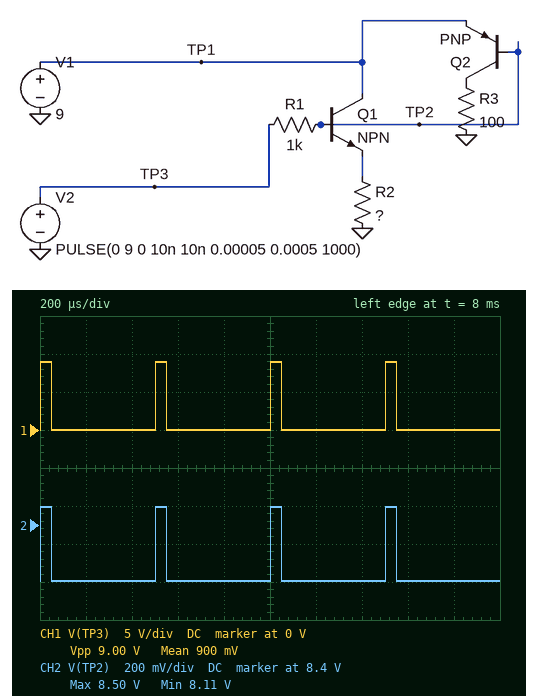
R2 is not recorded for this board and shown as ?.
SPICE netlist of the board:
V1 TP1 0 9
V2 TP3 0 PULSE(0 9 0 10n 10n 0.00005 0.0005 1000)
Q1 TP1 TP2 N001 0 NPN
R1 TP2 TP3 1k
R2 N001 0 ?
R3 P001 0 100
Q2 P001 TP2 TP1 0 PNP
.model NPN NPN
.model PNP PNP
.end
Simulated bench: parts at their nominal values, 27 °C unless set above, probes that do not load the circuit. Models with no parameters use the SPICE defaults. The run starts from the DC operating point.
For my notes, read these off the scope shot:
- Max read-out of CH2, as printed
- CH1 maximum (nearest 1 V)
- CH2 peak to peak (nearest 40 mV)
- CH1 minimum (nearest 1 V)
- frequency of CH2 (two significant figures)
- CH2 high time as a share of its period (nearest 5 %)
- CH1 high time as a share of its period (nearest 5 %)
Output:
8.50 V
9 V
400 mV
0 V
2.0 kHz
10 %
10 %
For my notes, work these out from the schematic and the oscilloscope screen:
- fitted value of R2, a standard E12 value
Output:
150 Ω
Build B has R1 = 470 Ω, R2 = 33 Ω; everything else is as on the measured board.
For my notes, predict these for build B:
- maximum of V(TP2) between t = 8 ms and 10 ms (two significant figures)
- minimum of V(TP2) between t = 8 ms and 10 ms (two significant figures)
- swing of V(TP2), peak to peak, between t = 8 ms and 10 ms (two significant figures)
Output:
8.1 V
8.1 V
35 mV
